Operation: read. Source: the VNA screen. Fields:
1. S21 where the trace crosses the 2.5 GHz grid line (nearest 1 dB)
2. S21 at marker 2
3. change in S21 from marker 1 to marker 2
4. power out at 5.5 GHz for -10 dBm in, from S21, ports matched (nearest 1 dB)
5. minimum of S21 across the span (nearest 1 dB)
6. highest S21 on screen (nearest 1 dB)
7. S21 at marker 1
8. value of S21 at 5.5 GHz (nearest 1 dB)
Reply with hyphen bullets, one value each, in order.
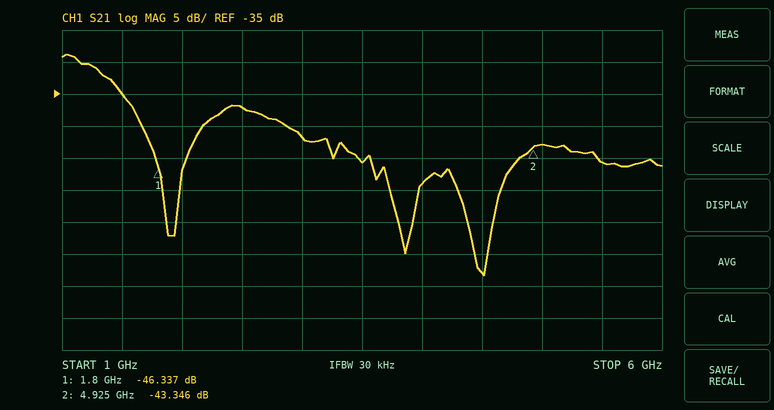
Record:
- -37 dB
- -43.346 dB
- 2.991 dB
- -56 dBm
- -63 dB
- -29 dB
- -46.337 dB
- -46 dB
